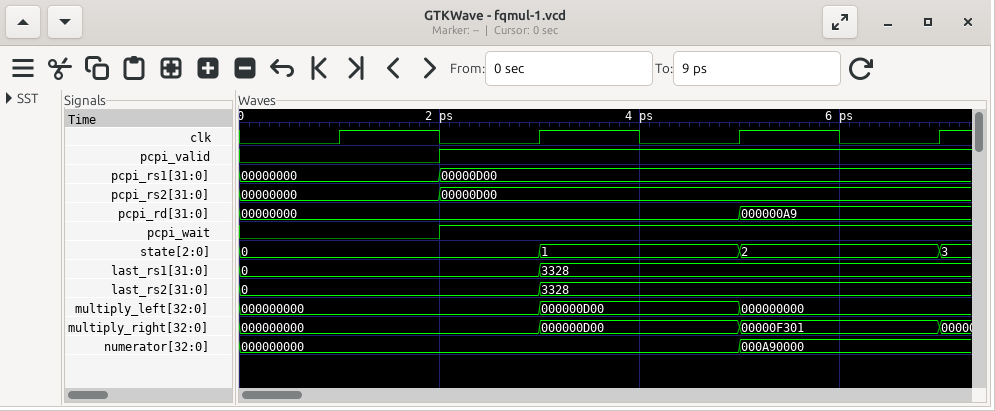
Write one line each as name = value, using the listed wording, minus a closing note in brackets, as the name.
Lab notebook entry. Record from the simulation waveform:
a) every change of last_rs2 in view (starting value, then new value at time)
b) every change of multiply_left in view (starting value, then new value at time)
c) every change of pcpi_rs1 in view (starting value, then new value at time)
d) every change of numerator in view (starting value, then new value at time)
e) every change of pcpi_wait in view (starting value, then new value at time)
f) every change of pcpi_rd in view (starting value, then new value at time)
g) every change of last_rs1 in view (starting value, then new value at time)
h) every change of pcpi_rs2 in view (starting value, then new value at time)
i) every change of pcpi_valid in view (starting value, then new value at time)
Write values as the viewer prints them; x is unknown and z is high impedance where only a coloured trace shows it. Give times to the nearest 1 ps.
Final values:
every change of last_rs2 in view = 0, 3328 at 3 ps
every change of multiply_left in view = 000000000, 000000D00 at 3 ps, 000000000 at 5 ps
every change of pcpi_rs1 in view = 00000000, 00000D00 at 2 ps
every change of numerator in view = 000000000, 000A90000 at 5 ps
every change of pcpi_wait in view = 0, 1 at 2 ps
every change of pcpi_rd in view = 00000000, 000000A9 at 5 ps
every change of last_rs1 in view = 0, 3328 at 3 ps
every change of pcpi_rs2 in view = 00000000, 00000D00 at 2 ps
every change of pcpi_valid in view = 0, 1 at 2 ps
